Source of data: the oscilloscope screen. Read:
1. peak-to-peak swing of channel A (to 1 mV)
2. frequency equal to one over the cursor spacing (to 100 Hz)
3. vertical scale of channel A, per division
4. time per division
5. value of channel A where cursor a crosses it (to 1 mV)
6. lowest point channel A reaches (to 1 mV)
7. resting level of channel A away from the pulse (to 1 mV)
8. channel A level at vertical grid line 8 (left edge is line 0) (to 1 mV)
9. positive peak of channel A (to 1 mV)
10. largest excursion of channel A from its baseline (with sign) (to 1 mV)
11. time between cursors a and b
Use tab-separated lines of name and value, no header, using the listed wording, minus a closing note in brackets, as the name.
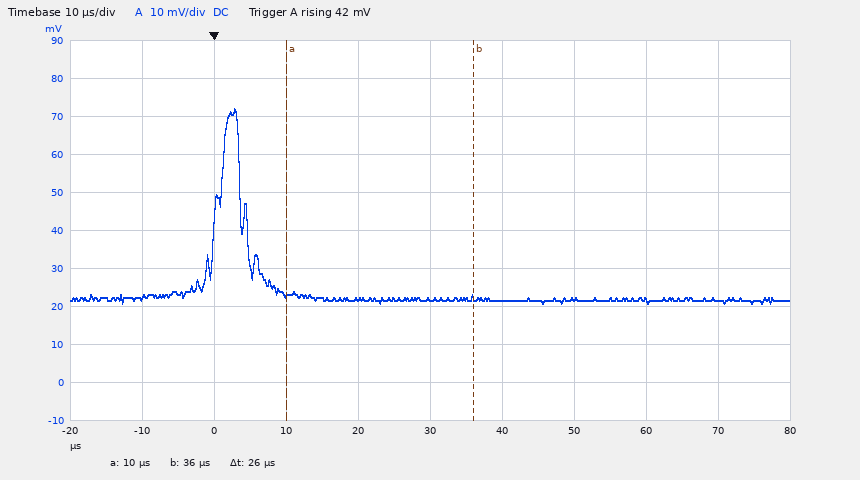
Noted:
peak-to-peak swing of channel A	51 mV
frequency equal to one over the cursor spacing	38.5 kHz
vertical scale of channel A, per division	10 mV
time per division	10 µs
value of channel A where cursor a crosses it	23 mV
lowest point channel A reaches	21 mV
resting level of channel A away from the pulse	22 mV
channel A level at vertical grid line 8 (left edge is line 0)	22 mV
positive peak of channel A	72 mV
largest excursion of channel A from its baseline (with sign)	+50 mV
time between cursors a and b	26 µs
